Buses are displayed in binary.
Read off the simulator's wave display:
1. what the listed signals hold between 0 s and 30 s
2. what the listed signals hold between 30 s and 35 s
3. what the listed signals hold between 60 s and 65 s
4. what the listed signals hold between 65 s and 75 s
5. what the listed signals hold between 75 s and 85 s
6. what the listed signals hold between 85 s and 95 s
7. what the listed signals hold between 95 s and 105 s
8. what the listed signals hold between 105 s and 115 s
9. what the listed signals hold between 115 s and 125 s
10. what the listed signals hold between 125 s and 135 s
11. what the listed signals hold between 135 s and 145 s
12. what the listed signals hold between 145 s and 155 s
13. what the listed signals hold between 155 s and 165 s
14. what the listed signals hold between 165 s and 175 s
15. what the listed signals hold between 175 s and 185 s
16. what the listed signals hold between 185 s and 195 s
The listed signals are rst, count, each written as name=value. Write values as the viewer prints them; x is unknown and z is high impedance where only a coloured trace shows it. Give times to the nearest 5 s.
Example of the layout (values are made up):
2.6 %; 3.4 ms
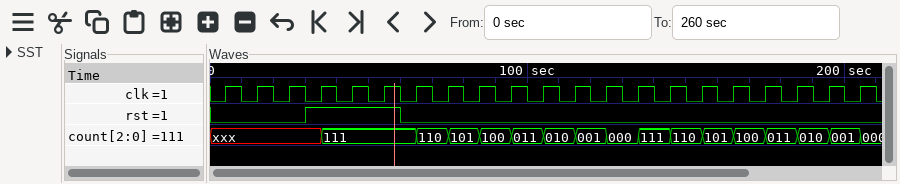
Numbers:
rst=0, count=xxx; rst=1, count=xxx; rst=0, count=111; rst=0, count=110; rst=0, count=101; rst=0, count=100; rst=0, count=011; rst=0, count=010; rst=0, count=001; rst=0, count=000; rst=0, count=111; rst=0, count=110; rst=0, count=101; rst=0, count=100; rst=0, count=011; rst=0, count=010
